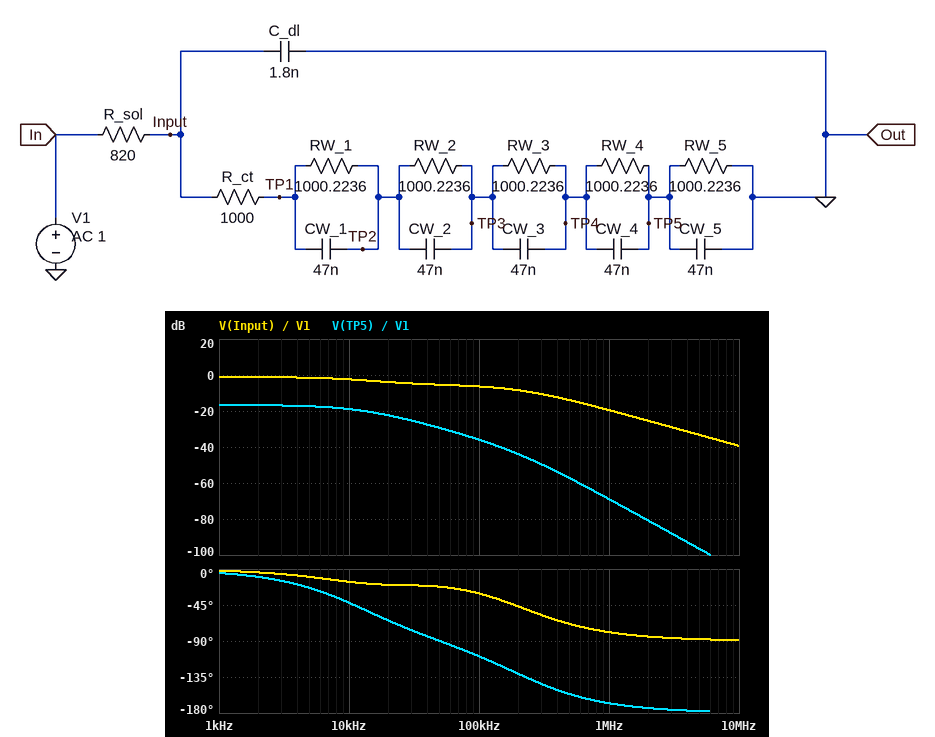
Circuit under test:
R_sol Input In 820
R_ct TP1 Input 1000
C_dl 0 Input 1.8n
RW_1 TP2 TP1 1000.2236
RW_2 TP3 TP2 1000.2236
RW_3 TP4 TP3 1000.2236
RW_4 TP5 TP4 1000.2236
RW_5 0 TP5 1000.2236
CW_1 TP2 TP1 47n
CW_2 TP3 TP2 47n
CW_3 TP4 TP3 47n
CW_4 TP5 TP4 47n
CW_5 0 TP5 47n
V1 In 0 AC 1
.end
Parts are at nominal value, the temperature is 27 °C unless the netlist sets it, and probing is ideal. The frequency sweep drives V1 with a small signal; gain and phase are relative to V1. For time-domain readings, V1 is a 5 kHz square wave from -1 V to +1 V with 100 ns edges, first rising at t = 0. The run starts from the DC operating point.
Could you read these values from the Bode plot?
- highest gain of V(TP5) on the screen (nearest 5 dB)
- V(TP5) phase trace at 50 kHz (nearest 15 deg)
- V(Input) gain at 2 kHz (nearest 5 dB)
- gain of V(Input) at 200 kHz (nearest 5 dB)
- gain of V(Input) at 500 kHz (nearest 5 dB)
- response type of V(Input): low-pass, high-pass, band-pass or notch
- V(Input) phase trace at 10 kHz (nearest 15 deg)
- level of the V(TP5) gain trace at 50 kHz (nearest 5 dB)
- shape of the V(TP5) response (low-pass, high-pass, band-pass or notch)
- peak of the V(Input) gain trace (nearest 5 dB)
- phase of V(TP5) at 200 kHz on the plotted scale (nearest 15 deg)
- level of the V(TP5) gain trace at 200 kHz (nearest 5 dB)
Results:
-15 dB
-90 deg
0 dB
-10 dB
-15 dB
low-pass
-15 deg
-30 dB
low-pass
0 dB
-135 deg
-45 dB
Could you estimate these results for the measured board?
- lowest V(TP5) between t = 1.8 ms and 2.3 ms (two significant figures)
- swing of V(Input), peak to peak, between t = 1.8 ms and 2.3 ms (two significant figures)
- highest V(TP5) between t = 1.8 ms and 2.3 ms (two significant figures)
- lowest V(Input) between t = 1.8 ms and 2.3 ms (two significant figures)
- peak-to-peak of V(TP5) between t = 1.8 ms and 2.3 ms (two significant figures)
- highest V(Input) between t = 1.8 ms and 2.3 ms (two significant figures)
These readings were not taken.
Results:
-150 mV
1.8 V
150 mV
-880 mV
290 mV
880 mV
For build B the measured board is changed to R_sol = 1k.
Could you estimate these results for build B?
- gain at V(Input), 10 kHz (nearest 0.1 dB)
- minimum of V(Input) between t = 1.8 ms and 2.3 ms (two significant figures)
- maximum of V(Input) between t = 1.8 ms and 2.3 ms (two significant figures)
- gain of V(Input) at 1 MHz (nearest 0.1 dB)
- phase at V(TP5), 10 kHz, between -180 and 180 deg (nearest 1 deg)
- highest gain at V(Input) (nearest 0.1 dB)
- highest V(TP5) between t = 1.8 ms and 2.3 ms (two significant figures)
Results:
-2.9 dB
-860 mV
860 mV
-21.2 dB
-45 deg
-1.3 dB
140 mV
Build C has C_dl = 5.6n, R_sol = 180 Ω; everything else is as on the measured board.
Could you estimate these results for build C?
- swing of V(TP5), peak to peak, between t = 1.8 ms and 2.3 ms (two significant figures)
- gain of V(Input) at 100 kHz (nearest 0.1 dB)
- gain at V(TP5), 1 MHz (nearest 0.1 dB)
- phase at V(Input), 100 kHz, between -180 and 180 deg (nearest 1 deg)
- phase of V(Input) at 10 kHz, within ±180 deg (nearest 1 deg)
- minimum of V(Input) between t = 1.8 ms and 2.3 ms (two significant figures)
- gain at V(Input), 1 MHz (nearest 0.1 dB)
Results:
320 mV
-2.6 dB
-65.6 dB
-29 deg
-7 deg
-970 mV
-16.2 dB
